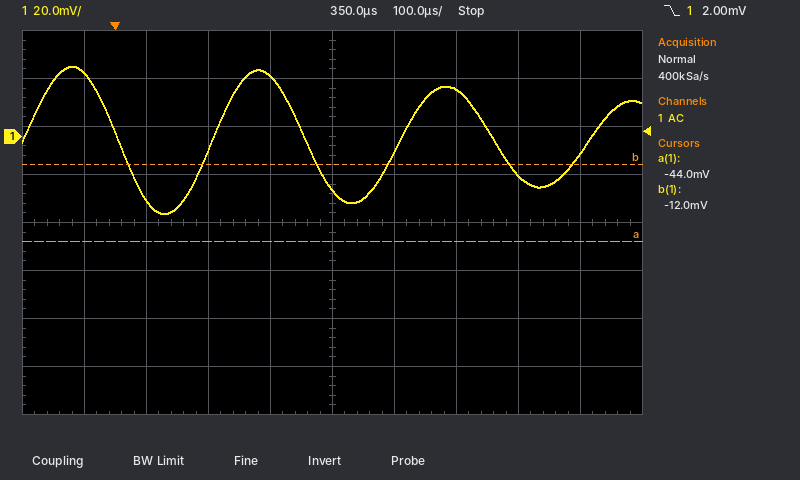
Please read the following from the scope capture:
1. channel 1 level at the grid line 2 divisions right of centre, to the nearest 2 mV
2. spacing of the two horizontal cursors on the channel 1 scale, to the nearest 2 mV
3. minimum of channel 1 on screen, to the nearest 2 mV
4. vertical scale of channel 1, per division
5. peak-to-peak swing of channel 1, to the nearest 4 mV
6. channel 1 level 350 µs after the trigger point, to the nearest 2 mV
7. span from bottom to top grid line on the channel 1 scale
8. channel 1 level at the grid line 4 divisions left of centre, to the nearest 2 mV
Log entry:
20 mV
32 mV
-32 mV
20 mV
60 mV
-22 mV
160 mV
26 mV
